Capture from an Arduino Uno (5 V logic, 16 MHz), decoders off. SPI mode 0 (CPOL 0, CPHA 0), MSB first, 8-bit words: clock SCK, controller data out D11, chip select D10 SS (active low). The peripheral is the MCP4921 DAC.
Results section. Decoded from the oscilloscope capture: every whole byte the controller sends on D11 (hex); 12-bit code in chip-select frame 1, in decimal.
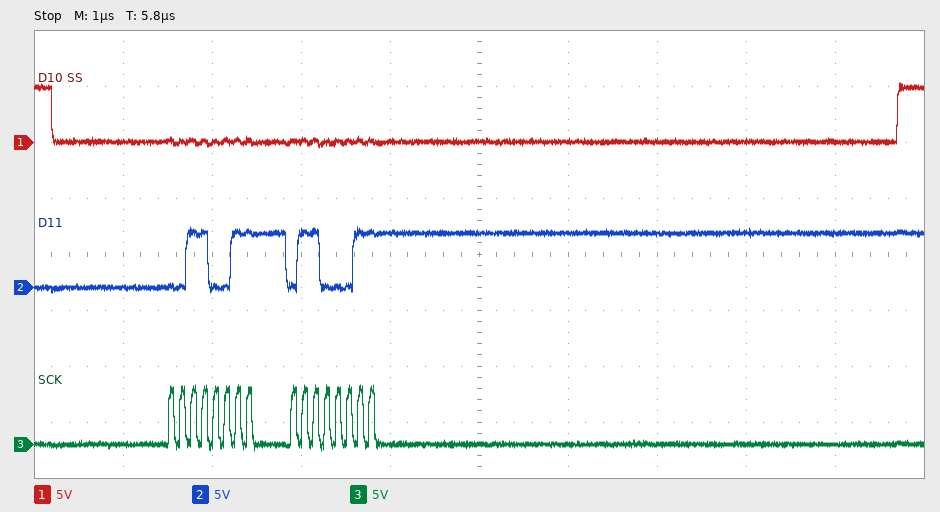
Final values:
33 63
867
